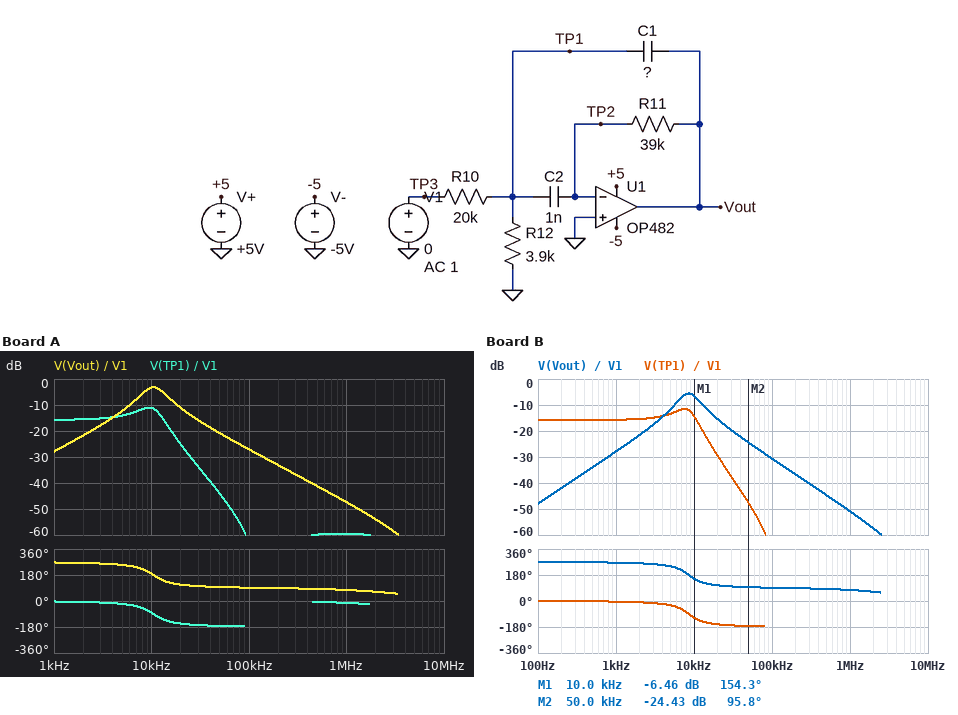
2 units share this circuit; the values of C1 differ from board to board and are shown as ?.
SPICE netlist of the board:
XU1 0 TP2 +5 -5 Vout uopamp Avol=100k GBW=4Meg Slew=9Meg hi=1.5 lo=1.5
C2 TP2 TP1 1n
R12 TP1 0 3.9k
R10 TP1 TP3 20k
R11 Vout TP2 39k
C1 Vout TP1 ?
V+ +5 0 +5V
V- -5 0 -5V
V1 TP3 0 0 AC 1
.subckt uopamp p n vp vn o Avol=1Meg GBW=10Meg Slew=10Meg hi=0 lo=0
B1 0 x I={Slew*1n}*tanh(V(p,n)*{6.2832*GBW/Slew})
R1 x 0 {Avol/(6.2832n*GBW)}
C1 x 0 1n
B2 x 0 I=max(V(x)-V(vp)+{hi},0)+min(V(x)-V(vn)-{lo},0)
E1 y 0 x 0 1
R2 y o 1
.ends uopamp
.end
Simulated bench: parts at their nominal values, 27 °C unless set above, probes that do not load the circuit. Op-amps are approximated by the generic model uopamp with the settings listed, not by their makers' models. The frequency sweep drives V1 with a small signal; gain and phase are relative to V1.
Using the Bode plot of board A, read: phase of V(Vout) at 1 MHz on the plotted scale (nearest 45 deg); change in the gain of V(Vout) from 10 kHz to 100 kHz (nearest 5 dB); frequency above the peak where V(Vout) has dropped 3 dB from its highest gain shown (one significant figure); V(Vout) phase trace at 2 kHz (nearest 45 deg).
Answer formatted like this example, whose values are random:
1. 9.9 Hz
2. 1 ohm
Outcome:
1. 90 deg
2. -25 dB
3. 10 kHz
4. 270 deg
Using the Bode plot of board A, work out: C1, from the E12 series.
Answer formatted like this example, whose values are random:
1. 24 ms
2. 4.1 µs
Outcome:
1. 1.8 nF
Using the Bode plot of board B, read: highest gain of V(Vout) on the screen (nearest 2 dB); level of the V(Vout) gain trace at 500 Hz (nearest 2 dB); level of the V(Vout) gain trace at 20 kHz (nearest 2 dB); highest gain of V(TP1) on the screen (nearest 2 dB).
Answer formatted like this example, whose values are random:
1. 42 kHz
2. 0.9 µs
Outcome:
1. -6 dB
2. -34 dB
3. -16 dB
4. -12 dB
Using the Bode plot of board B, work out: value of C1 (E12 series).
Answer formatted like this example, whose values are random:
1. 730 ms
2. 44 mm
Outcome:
1. 2.7 nF
